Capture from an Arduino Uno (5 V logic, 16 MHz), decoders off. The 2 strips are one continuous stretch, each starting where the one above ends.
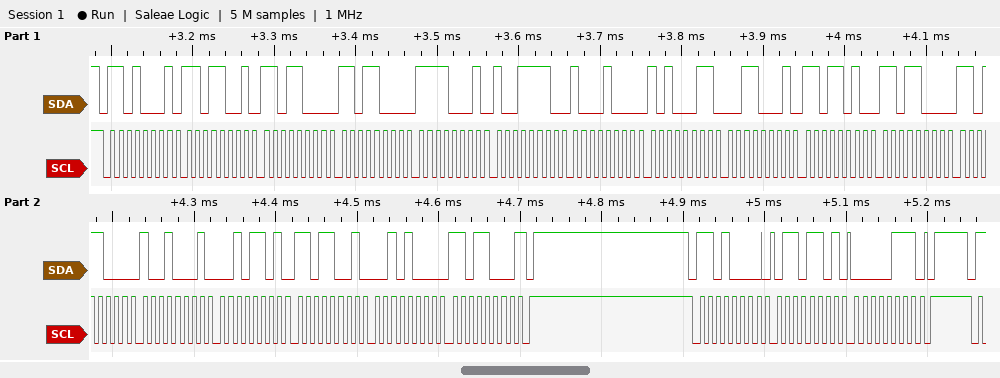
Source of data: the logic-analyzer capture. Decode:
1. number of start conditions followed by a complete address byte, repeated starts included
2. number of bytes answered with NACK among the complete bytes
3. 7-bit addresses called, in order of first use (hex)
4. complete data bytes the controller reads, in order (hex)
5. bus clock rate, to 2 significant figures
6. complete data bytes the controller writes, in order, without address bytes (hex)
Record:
2
1
0x68
D9 D8 D8 F1 9E 88 A3 31 DA D8 D8 91 2D D9 28 D8
100 kHz
6D 07
